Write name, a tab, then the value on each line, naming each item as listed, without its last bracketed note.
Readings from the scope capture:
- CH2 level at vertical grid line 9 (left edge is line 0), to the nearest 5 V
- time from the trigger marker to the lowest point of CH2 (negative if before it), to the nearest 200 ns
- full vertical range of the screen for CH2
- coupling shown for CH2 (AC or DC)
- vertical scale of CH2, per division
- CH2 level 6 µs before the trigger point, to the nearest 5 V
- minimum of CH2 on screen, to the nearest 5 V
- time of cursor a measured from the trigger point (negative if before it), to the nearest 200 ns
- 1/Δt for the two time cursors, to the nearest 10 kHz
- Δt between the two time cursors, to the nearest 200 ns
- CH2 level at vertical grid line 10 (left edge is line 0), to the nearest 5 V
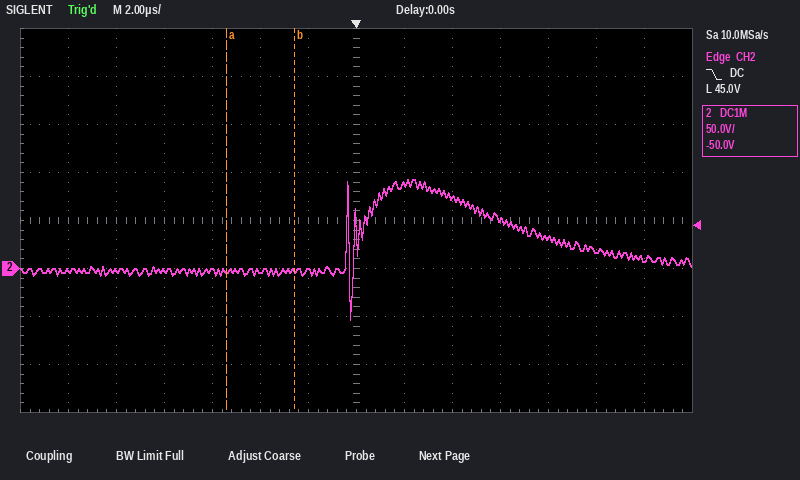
CH2 level at vertical grid line 9 (left edge is line 0), to the nearest 5 V	75 V
time from the trigger marker to the lowest point of CH2 (negative if before it), to the nearest 200 ns	-200 ns
full vertical range of the screen for CH2	400 V
coupling shown for CH2	DC
vertical scale of CH2, per division	50 V
CH2 level 6 µs before the trigger point, to the nearest 5 V	0 V
minimum of CH2 on screen, to the nearest 5 V	-55 V
time of cursor a measured from the trigger point (negative if before it), to the nearest 200 ns	-5.4 µs
1/Δt for the two time cursors, to the nearest 10 kHz	360 kHz
Δt between the two time cursors, to the nearest 200 ns	2.8 µs
CH2 level at vertical grid line 10 (left edge is line 0), to the nearest 5 V	50 V
